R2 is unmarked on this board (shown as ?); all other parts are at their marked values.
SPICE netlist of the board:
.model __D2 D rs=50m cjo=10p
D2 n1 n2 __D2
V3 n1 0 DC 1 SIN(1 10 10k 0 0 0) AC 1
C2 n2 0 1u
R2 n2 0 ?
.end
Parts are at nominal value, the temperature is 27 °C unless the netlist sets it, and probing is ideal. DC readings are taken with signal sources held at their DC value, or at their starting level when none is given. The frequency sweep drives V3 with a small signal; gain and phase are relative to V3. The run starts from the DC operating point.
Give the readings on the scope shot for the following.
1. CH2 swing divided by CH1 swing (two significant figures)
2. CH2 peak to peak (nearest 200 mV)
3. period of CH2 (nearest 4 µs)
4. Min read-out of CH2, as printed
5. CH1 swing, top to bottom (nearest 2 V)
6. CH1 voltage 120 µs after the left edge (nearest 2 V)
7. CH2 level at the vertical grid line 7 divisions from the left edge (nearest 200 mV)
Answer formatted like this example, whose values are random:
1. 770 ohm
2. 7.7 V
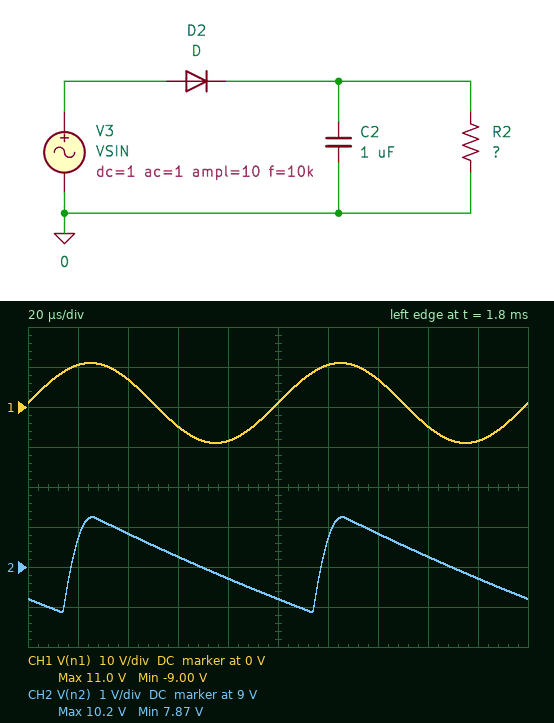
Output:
1. 0.12
2. 2.4 V
3. 100 µs
4. 7.87 V
5. 20 V
6. 10 V
7. 9.8 V
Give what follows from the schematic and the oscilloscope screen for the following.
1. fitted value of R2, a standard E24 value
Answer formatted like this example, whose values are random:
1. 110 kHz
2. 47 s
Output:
1. 330 Ω
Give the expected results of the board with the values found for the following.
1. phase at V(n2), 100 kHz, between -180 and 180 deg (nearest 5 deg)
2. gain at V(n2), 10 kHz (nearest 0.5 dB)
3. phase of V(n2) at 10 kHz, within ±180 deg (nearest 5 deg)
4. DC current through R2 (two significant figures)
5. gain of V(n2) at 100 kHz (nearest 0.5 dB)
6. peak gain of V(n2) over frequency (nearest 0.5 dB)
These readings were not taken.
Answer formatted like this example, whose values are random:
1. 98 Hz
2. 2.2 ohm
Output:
1. -85 deg
2. -5.5 dB
3. -55 deg
4. 1.0 mA
5. -24.0 dB
6. -0.5 dB
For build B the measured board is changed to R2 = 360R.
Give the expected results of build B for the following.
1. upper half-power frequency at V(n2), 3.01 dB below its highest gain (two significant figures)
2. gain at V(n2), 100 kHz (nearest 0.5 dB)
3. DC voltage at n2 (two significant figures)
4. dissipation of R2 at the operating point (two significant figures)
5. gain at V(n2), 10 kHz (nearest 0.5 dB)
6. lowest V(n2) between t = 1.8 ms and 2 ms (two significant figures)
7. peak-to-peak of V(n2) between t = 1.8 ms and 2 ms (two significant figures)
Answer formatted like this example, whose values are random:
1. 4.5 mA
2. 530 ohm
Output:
1. 6.3 kHz
2. -24.5 dB
3. 350 mV
4. 330 µW
5. -6.0 dB
6. 8.0 V
7. 2.2 V
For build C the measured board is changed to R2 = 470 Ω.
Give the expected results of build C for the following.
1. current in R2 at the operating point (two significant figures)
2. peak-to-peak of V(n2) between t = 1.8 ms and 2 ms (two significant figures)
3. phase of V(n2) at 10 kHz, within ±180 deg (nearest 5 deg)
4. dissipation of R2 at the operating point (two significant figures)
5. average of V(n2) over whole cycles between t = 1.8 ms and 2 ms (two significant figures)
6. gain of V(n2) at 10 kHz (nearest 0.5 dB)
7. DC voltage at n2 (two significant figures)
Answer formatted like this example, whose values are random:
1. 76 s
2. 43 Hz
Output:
1. 750 µA
2. 1.8 V
3. -65 deg
4. 260 µW
5. 9.4 V
6. -7.5 dB
7. 350 mV
